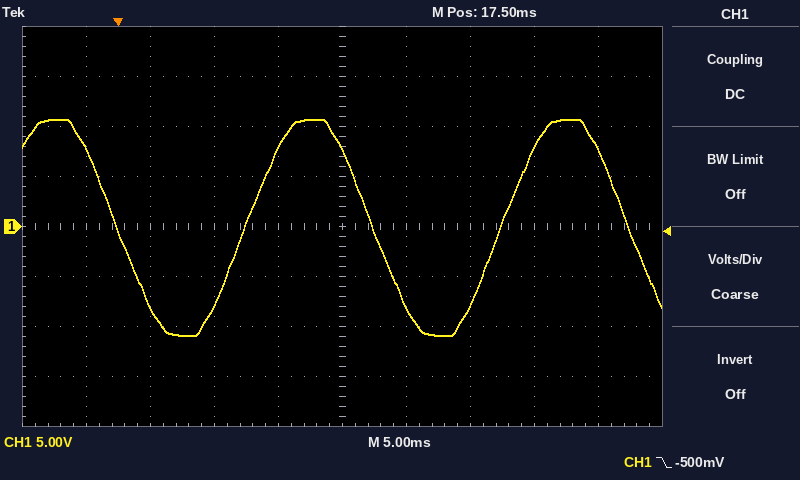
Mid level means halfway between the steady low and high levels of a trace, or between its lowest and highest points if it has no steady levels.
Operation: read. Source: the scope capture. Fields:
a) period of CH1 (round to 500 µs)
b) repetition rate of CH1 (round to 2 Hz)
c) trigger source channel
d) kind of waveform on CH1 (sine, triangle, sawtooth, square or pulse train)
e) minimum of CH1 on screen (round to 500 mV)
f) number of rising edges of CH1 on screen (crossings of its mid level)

20.0 ms
50 Hz
CH1
sine
-11.0 V
2
